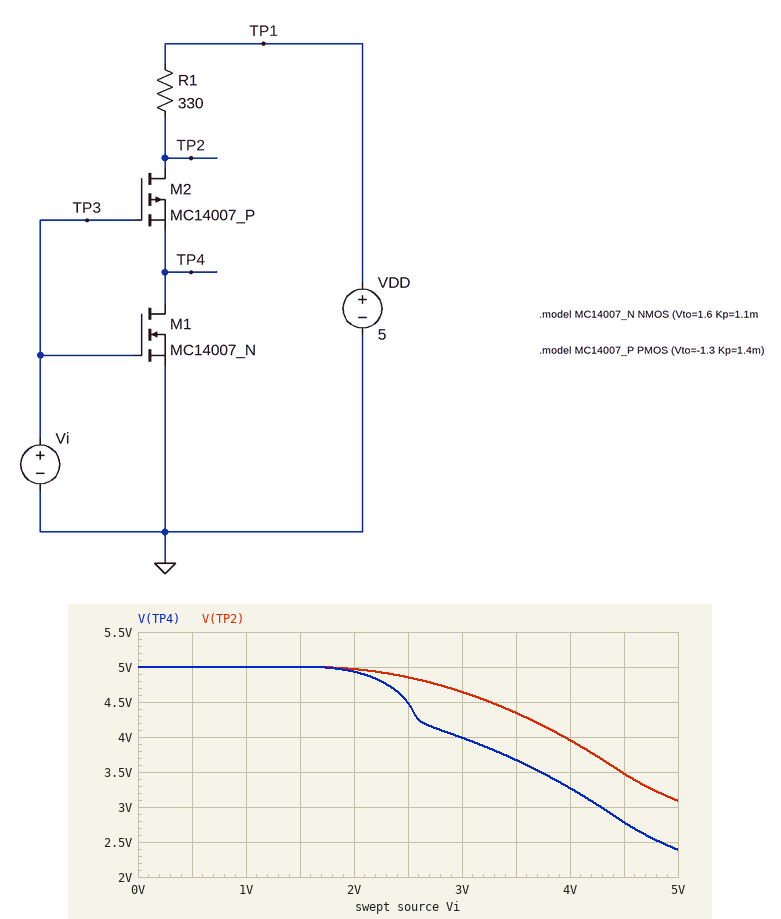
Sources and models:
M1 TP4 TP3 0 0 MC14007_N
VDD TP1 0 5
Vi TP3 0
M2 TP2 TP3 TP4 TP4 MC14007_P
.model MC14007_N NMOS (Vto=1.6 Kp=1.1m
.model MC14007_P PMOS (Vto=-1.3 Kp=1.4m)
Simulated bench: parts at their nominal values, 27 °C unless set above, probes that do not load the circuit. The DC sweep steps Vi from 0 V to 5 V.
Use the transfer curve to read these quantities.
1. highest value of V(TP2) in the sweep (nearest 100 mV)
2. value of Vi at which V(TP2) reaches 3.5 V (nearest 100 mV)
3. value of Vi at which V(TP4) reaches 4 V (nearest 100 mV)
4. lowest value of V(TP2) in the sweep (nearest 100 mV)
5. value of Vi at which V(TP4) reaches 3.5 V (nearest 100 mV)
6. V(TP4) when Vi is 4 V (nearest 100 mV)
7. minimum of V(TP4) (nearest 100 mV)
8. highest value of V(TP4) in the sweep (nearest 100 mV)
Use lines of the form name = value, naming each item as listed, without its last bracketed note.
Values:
highest value of V(TP2) in the sweep = 5.0 V
value of Vi at which V(TP2) reaches 3.5 V = 4.5 V
value of Vi at which V(TP4) reaches 4 V = 3.0 V
lowest value of V(TP2) in the sweep = 3.1 V
value of Vi at which V(TP4) reaches 3.5 V = 3.7 V
V(TP4) when Vi is 4 V = 3.3 V
minimum of V(TP4) = 2.4 V
highest value of V(TP4) in the sweep = 5.0 V
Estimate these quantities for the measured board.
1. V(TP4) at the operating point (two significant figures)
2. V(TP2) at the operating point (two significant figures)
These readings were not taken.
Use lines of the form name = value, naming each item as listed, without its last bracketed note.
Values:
V(TP4) at the operating point = 5.0 V
V(TP2) at the operating point = 5.0 V
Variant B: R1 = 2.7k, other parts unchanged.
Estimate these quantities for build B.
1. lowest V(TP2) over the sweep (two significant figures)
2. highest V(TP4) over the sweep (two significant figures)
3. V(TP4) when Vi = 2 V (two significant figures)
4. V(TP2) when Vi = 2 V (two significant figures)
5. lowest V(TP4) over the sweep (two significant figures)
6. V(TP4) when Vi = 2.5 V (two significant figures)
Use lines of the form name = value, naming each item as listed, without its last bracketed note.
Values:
lowest V(TP2) over the sweep = 1.1 V
highest V(TP4) over the sweep = 5.0 V
V(TP4) when Vi = 2 V = 4.7 V
V(TP2) when Vi = 2 V = 4.8 V
lowest V(TP4) over the sweep = 410 mV
V(TP4) when Vi = 2.5 V = 3.2 V
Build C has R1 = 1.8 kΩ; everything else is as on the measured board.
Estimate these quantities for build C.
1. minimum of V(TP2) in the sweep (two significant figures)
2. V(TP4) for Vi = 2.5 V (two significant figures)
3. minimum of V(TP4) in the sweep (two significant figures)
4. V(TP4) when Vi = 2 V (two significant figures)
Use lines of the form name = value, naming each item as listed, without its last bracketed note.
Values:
minimum of V(TP2) in the sweep = 1.3 V
V(TP4) for Vi = 2.5 V = 3.6 V
minimum of V(TP4) in the sweep = 610 mV
V(TP4) when Vi = 2 V = 4.8 V
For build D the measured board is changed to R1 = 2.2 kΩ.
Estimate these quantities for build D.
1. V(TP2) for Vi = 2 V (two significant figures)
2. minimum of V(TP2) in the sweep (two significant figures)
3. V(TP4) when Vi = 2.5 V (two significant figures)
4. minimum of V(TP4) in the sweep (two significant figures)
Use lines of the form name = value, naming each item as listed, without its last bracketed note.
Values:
V(TP2) for Vi = 2 V = 4.8 V
minimum of V(TP2) in the sweep = 1.2 V
V(TP4) when Vi = 2.5 V = 3.4 V
minimum of V(TP4) in the sweep = 500 mV
